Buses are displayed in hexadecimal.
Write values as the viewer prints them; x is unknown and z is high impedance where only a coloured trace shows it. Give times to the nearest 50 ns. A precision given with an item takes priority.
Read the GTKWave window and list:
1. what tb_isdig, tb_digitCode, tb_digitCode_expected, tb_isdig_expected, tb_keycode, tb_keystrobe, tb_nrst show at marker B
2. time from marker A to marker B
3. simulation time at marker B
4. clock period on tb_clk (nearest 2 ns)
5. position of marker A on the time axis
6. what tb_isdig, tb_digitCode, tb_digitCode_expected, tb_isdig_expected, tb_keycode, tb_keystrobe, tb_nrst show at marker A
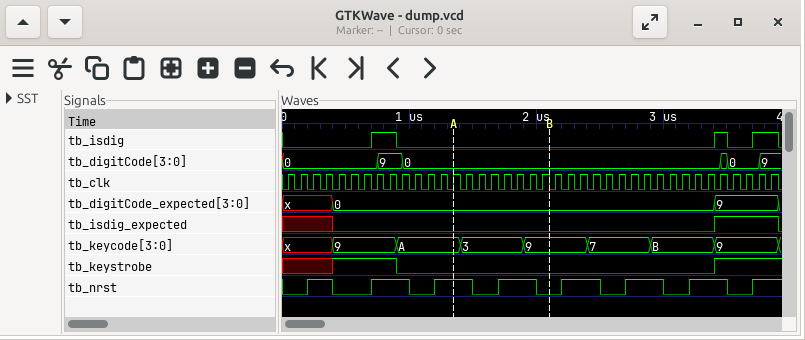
tb_isdig=0, tb_digitCode=0, tb_digitCode_expected=0, tb_isdig_expected=0, tb_keycode=9, tb_keystrobe=0, tb_nrst=0
750 ns
2100 ns
100 ns
1350 ns
tb_isdig=0, tb_digitCode=0, tb_digitCode_expected=0, tb_isdig_expected=0, tb_keycode=A, tb_keystrobe=0, tb_nrst=1
